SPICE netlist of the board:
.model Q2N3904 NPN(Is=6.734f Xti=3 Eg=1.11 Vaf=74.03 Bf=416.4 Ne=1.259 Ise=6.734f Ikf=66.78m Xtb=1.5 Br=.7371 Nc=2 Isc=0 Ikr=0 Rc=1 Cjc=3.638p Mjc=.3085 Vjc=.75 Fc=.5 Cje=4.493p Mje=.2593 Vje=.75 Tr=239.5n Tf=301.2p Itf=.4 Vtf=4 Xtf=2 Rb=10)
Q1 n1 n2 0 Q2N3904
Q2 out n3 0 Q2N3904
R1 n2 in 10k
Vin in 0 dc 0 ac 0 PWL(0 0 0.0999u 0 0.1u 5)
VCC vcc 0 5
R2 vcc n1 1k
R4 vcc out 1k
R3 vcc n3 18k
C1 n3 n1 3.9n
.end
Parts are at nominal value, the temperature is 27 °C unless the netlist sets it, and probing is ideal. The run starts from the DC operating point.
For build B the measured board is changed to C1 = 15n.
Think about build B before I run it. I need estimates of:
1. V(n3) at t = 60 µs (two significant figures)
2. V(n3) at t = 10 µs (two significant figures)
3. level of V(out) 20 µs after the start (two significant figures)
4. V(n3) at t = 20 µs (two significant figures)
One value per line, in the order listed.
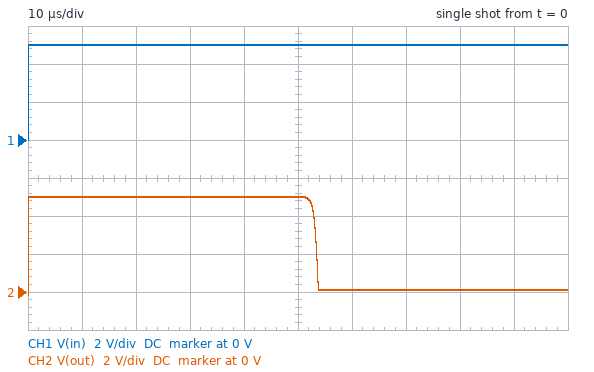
-2.4 V
-3.9 V
5.0 V
-3.5 V
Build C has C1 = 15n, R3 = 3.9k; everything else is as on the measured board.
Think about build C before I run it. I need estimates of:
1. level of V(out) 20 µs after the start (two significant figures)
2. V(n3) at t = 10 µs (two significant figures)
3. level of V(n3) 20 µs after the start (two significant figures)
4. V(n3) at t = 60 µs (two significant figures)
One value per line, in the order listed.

5.0 V
-2.7 V
-1.5 V
730 mV
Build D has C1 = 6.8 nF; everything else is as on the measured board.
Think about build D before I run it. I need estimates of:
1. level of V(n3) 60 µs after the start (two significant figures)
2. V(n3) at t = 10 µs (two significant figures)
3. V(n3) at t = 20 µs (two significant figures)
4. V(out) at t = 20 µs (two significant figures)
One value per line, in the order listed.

-640 mV
-3.5 V
-2.8 V
5.0 V
